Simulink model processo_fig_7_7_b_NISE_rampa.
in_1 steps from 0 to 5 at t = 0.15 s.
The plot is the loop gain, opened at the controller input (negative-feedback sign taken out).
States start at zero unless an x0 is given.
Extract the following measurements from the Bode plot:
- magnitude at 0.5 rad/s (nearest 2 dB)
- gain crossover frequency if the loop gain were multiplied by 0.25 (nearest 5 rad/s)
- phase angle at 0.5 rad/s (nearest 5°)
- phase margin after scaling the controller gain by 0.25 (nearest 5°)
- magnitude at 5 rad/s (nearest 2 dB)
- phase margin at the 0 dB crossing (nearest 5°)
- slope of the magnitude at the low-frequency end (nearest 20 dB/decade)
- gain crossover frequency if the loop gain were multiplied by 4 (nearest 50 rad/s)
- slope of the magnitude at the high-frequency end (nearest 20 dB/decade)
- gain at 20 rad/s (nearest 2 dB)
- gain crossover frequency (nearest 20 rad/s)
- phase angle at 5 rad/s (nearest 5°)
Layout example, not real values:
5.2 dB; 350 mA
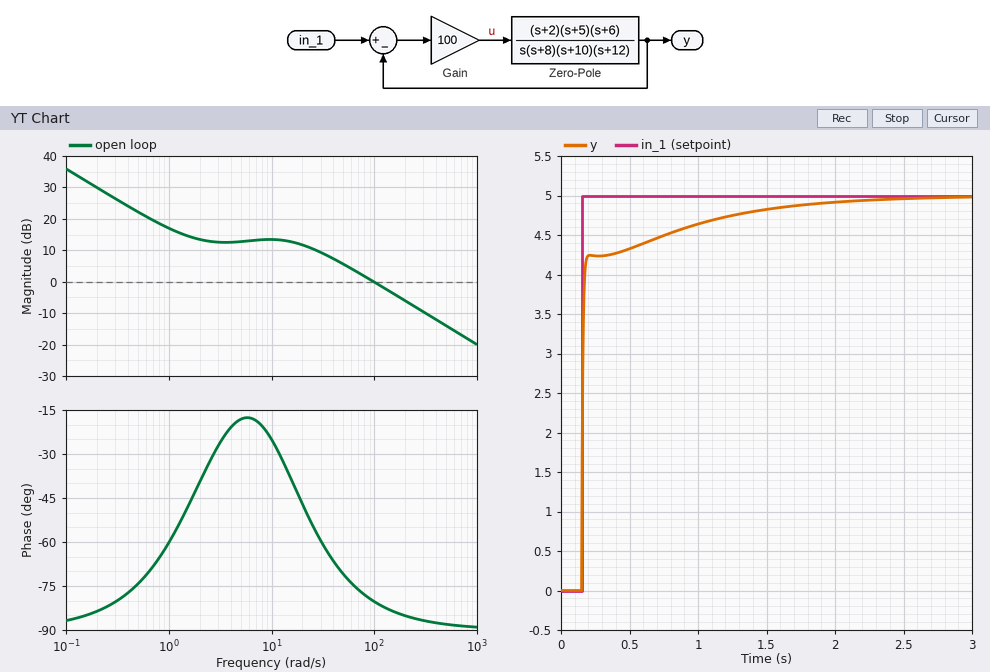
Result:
22 dB; 20 rad/s; -75°; 135°; 12 dB; 100°; -20 dB/decade; 400 rad/s; -20 dB/decade; 12 dB; 100 rad/s; -20°
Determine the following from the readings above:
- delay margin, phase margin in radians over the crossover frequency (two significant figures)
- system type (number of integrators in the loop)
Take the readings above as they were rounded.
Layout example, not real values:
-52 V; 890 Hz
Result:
0.017 s; 1
